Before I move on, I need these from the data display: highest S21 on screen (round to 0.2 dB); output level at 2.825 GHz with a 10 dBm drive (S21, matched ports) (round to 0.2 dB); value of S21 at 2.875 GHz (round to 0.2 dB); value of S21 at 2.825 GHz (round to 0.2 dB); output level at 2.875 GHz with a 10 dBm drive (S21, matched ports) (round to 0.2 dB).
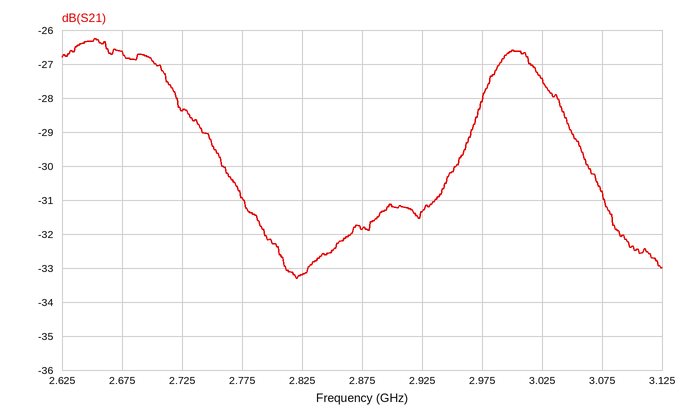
-26.2 dB
-23.2 dBm
-31.8 dB
-33.2 dB
-21.8 dBm
